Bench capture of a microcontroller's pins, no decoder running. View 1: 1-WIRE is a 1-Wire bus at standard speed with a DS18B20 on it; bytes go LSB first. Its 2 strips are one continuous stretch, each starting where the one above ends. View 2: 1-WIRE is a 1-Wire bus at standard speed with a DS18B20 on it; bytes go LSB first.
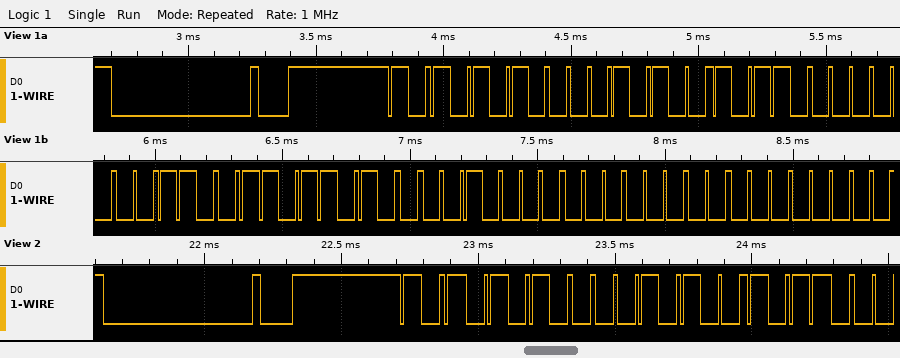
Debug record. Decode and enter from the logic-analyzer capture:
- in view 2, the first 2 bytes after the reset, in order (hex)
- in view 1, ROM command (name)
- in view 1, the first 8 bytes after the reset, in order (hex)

55 28
Match ROM
55 28 0D 30 5B 08 00 00
